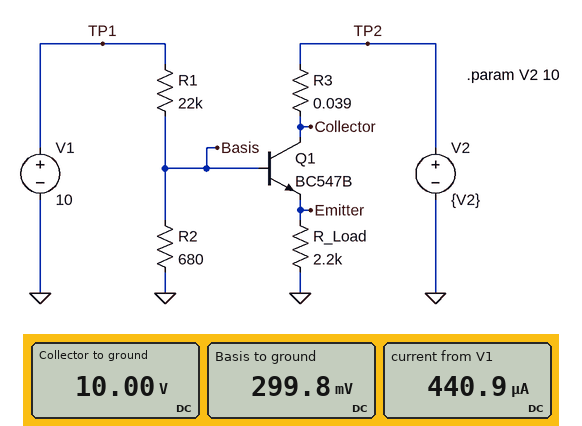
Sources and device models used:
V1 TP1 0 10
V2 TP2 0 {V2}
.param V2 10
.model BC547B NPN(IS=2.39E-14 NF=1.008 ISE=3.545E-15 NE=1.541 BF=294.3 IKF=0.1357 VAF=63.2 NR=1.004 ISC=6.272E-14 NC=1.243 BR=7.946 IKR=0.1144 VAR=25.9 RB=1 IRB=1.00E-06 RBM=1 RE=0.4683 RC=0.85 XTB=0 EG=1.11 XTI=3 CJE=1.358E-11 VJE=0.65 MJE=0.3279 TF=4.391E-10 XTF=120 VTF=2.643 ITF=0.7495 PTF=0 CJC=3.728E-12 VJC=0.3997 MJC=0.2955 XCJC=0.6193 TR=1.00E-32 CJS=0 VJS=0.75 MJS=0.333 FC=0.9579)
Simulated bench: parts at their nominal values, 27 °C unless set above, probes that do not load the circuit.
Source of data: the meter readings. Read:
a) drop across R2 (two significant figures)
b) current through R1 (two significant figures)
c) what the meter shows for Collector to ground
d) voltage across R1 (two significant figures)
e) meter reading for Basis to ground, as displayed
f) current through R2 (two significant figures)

300 mV
440 µA
10.00 V
9.7 V
299.8 mV
440 µA
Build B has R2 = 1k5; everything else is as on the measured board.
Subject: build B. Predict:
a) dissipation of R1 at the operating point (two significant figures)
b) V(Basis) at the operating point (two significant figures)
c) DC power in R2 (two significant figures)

4.0 mW
640 mV
270 µW
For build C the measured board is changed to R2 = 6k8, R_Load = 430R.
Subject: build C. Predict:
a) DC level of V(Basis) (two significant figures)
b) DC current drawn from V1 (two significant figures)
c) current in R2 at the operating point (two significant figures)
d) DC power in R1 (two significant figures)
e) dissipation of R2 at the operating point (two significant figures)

2.3 V
350 µA
340 µA
2.7 mW
780 µW
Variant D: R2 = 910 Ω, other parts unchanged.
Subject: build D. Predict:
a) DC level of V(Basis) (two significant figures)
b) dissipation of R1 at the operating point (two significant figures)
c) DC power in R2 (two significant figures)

400 mV
4.2 mW
170 µW
